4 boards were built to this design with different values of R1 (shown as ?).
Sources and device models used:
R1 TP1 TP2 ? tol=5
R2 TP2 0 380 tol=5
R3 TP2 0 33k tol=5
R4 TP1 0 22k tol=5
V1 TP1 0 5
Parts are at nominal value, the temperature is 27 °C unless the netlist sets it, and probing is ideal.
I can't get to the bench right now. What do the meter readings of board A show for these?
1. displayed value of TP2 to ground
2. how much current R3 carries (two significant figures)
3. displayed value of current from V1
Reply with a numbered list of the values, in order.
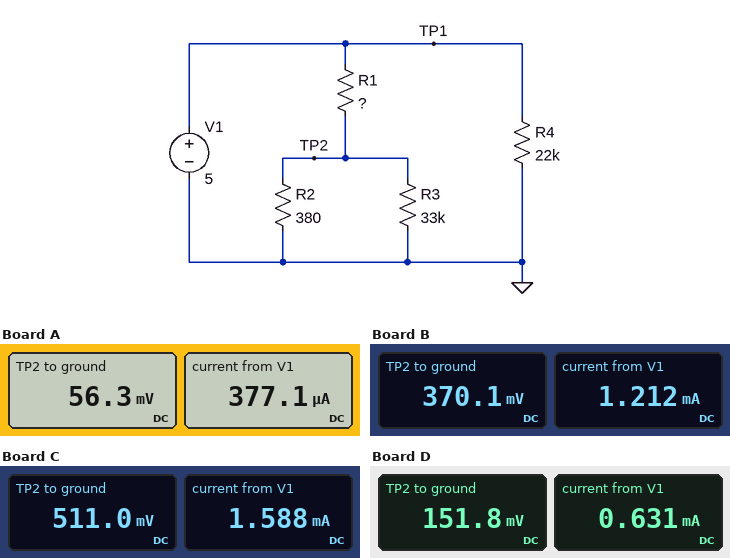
1. 56.3 mV
2. 1.7 µA
3. 377.1 µA
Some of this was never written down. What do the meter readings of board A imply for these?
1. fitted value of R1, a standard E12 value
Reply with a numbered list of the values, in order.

1. 33 kΩ
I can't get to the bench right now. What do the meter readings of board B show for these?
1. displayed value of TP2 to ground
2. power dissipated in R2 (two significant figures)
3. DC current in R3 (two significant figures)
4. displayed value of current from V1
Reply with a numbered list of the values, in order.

1. 370.1 mV
2. 360 µW
3. 11 µA
4. 1.212 mA
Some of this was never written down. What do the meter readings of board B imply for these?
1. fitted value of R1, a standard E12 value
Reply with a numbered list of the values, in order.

1. 4.7 kΩ
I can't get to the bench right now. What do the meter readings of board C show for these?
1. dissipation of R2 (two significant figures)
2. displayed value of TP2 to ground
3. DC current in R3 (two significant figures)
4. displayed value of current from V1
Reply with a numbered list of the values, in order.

1. 690 µW
2. 511.0 mV
3. 15 µA
4. 1.588 mA
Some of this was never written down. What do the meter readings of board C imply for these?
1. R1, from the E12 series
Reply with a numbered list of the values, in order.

1. 3.3 kΩ
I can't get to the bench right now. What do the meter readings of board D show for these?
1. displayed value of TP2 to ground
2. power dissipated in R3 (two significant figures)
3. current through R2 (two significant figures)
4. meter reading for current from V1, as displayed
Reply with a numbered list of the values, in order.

1. 151.8 mV
2. 700 nW
3. 400 µA
4. 0.631 mA
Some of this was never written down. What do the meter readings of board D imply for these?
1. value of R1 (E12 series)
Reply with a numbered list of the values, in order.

1. 12 kΩ
